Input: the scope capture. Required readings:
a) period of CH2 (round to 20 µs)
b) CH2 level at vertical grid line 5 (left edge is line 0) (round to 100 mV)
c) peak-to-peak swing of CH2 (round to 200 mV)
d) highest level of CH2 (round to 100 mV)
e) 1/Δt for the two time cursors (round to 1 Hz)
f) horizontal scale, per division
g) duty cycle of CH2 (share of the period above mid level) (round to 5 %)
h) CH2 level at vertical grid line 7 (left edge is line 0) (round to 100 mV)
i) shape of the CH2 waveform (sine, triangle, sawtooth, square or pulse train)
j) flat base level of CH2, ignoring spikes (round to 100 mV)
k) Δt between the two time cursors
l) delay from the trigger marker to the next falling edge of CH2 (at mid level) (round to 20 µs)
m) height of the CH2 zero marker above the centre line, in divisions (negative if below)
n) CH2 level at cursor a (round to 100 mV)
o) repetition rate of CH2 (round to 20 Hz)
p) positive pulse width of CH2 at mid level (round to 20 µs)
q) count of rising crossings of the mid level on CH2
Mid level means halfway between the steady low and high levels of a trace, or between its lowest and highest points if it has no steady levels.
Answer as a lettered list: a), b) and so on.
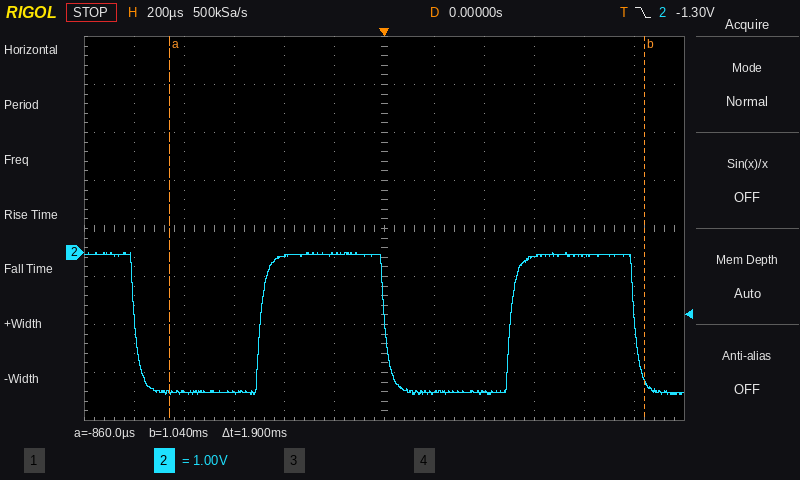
a) 1.00 ms
b) 0.0 V
c) 3.0 V
d) 0.0 V
e) 526 Hz
f) 200 µs
g) 50 %
h) -2.9 V
i) square
j) -2.9 V
k) 1.9 ms
l) 1.00 ms
m) -0.5 div
n) -2.9 V
o) 1.00 kHz
p) 500 µs
q) 2
